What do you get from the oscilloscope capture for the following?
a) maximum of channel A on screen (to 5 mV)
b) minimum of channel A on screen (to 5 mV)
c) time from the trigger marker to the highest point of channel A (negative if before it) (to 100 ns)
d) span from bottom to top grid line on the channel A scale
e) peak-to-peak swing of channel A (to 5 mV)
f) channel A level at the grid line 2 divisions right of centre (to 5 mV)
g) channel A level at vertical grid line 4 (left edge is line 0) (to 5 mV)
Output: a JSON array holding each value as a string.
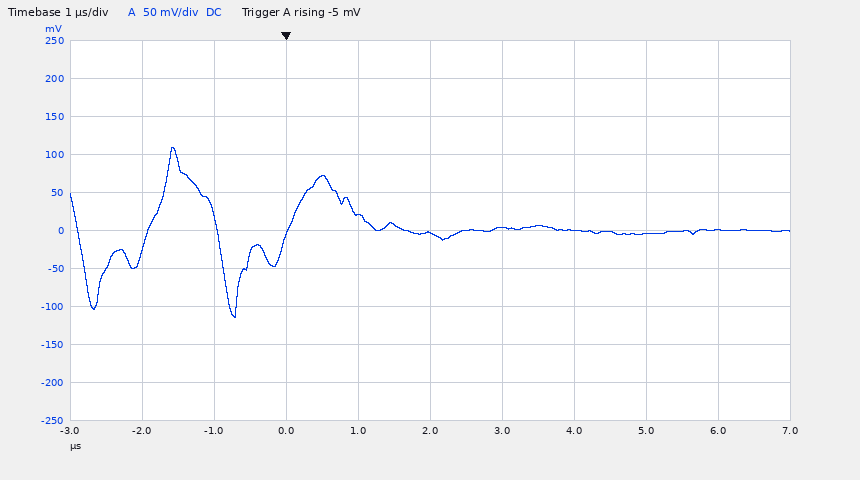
["110 mV", "-115 mV", "-1.6 µs", "500 mV", "225 mV", "0 mV", "20 mV"]
